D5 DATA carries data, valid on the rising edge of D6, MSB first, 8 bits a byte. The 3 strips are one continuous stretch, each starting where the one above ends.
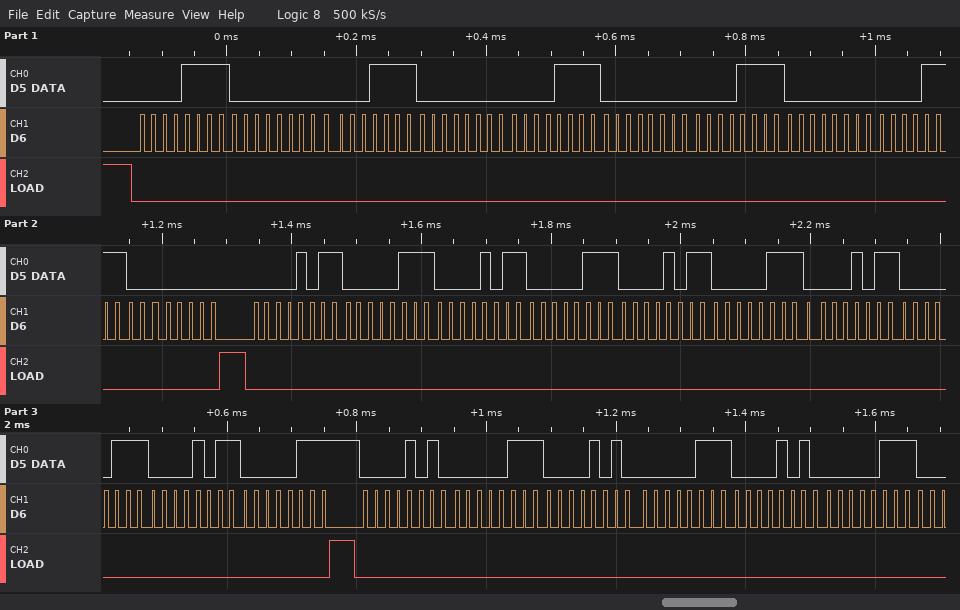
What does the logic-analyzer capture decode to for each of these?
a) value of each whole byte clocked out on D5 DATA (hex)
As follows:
0F 00 0F 00 0F 00 0F 00 0F 00 0B 07 0B 07 0B 07 0B 07 0B 07 0A 07 0A 07 0A 07
